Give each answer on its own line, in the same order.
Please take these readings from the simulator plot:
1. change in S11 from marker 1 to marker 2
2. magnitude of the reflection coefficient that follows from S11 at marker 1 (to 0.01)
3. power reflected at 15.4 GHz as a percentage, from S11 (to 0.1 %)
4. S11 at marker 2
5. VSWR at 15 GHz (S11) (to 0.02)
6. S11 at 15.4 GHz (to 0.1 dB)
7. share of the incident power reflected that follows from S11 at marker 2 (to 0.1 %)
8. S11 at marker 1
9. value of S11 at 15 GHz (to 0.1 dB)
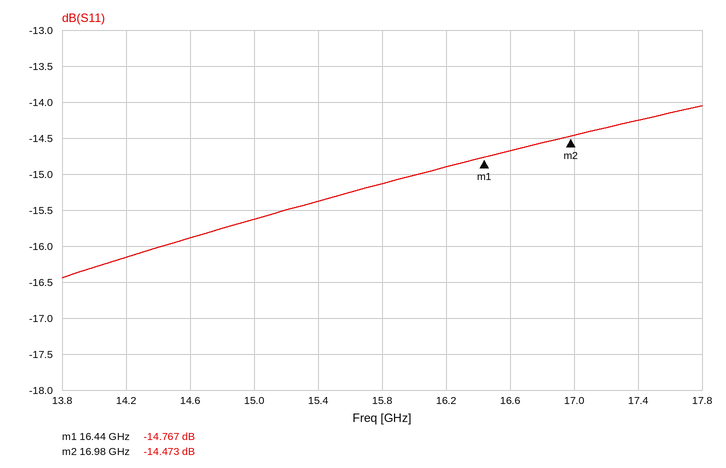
0.294 dB
0.18
2.9 %
-14.473 dB
1.40
-15.4 dB
3.6 %
-14.767 dB
-15.6 dB
